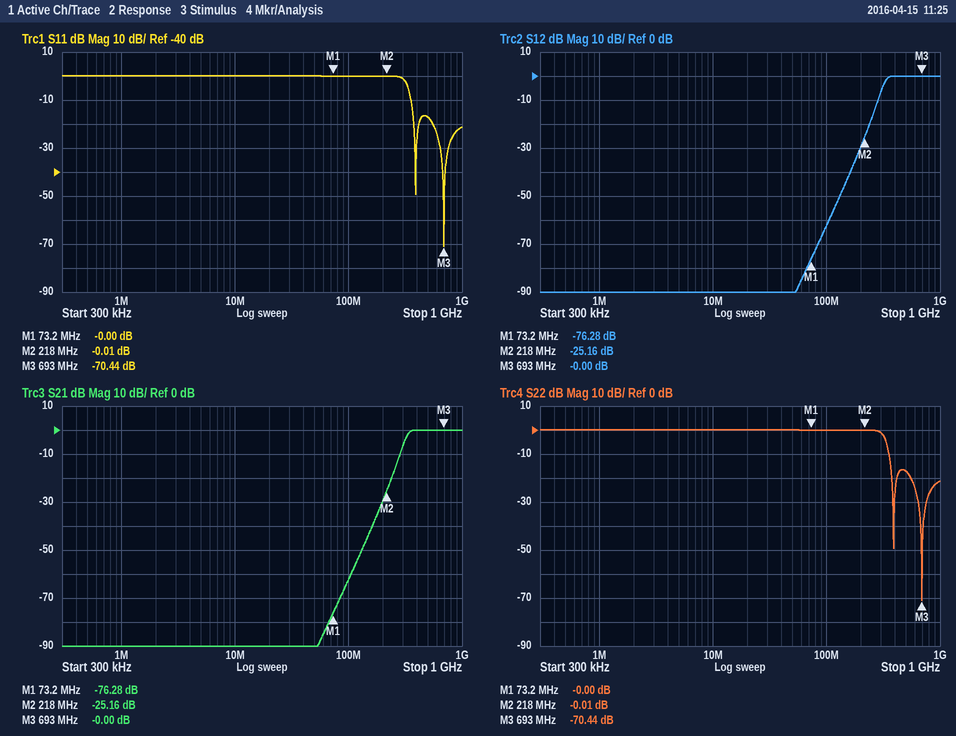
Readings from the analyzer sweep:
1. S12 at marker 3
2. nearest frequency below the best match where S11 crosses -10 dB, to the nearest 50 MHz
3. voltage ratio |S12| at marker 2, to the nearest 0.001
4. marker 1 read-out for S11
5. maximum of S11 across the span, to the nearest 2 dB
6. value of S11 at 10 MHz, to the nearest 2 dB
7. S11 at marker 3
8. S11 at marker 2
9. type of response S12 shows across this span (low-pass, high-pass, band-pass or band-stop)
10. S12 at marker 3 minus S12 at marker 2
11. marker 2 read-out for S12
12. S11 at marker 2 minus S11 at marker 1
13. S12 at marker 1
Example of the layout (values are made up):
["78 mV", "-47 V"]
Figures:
["-0.00 dB", "350 MHz", "0.055", "-0.00 dB", "0 dB", "0 dB", "-70.44 dB", "-0.01 dB", "high-pass", "25.16 dB", "-25.16 dB", "-0.01 dB", "-76.28 dB"]
